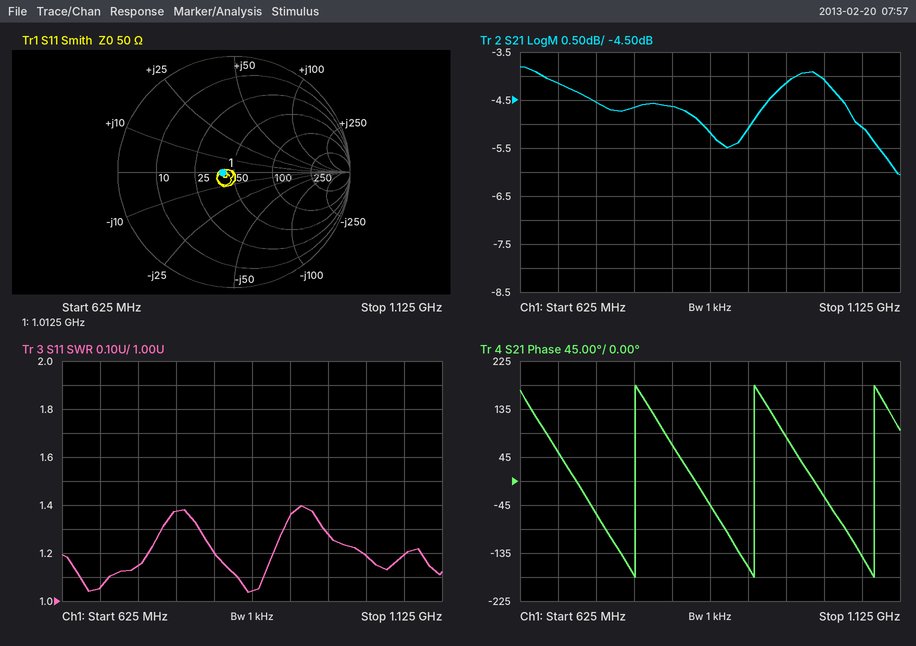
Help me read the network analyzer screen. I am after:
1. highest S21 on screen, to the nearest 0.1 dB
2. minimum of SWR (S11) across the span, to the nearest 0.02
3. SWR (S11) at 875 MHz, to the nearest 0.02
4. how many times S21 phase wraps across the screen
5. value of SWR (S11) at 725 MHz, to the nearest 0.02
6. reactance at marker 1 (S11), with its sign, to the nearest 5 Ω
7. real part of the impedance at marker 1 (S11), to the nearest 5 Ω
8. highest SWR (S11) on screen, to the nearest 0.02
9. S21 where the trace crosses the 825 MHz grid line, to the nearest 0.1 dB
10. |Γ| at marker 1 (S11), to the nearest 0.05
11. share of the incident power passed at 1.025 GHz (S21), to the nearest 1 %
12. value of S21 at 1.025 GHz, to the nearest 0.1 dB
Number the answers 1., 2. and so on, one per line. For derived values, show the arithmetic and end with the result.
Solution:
1. -3.8 dB
2. 1.04
3. 1.04
4. 3
5. 1.14
6. 0 Ω
7. 40 Ω
8. 1.40
9. -4.6 dB
10. 0.10
11. 10^(-4.1/10) ≈ 39 %
12. -4.1 dB
